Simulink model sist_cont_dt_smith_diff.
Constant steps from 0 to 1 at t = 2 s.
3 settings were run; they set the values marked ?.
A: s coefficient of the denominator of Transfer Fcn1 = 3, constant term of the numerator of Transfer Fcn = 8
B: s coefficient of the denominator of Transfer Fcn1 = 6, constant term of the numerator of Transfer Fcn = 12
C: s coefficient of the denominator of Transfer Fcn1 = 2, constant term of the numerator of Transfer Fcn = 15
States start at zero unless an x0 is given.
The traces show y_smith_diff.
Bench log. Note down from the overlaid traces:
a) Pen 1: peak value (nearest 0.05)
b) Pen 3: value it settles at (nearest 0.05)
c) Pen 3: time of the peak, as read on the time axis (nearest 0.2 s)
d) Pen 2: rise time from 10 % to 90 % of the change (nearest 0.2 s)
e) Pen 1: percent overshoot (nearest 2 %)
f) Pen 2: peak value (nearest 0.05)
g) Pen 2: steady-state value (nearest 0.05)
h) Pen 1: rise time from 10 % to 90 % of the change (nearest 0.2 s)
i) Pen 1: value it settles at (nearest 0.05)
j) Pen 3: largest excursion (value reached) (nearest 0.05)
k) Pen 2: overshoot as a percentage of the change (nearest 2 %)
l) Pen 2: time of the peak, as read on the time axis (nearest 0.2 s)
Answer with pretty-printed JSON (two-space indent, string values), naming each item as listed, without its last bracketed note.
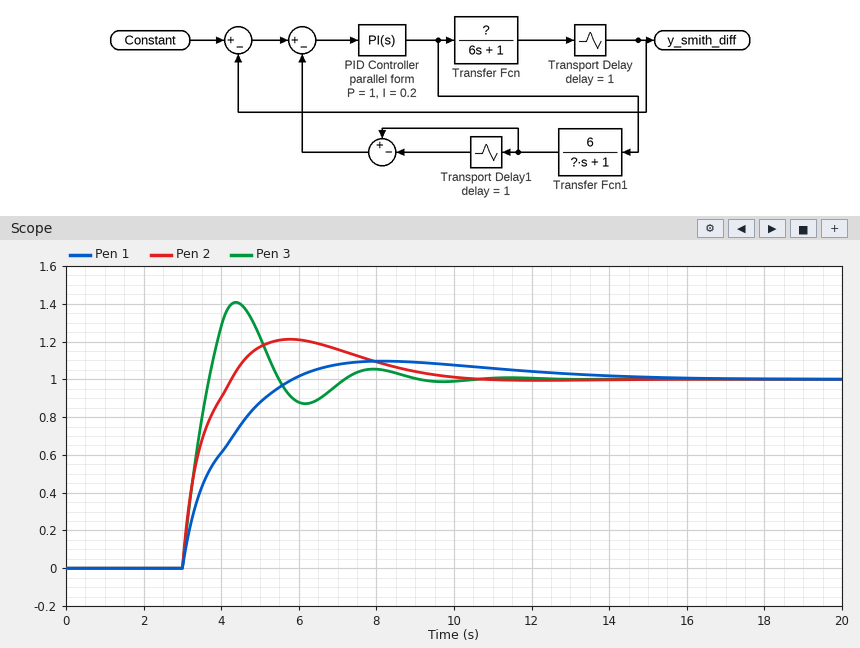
{
  "Pen 1: peak value": "1.10",
  "Pen 3: value it settles at": "1.00",
  "Pen 3: time of the peak, as read on the time axis": "4.4 s",
  "Pen 2: rise time from 10 % to 90 % of the change": "1.0 s",
  "Pen 1: percent overshoot": "10 %",
  "Pen 2: peak value": "1.20",
  "Pen 2: steady-state value": "1.00",
  "Pen 1: rise time from 10 % to 90 % of the change": "2.0 s",
  "Pen 1: value it settles at": "1.00",
  "Pen 3: largest excursion (value reached)": "1.40",
  "Pen 2: overshoot as a percentage of the change": "22 %",
  "Pen 2: time of the peak, as read on the time axis": "5.8 s"
}
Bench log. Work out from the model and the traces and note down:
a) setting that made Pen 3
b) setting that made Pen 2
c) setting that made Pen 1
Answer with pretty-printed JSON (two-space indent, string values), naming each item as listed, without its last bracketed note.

{
  "setting that made Pen 3": "B",
  "setting that made Pen 2": "C",
  "setting that made Pen 1": "A"
}
